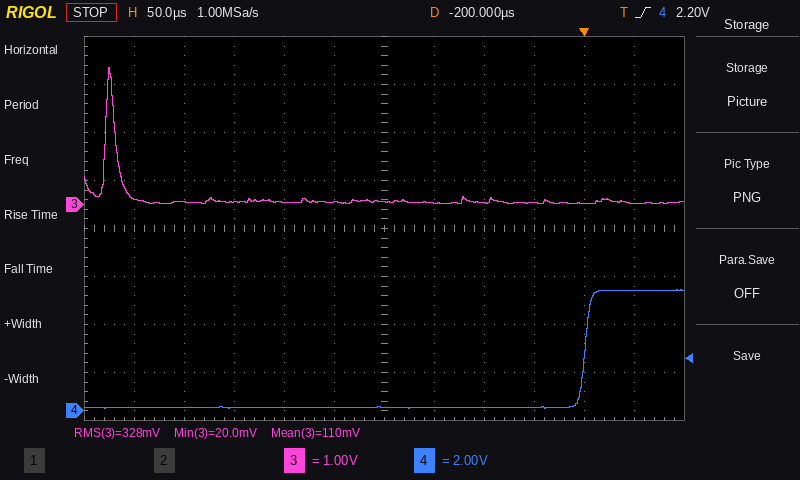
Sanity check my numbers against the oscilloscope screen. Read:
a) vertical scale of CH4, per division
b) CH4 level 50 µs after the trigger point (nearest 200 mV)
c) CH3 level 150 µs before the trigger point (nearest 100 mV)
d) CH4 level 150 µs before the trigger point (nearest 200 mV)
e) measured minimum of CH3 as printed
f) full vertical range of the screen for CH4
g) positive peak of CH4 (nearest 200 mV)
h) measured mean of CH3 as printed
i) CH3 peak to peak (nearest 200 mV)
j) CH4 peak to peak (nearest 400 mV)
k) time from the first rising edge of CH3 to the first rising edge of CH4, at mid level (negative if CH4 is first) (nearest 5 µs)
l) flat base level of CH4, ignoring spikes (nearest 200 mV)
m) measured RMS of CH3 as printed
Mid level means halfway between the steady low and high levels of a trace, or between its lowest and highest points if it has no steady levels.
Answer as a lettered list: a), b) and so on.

a) 2 V
b) 5.0 V
c) 0.0 V
d) 200 mV
e) 20.0 mV
f) 16 V
g) 5.0 V
h) 110 mV
i) 2.8 V
j) 4.8 V
k) +480 µs
l) 200 mV
m) 328 mV
